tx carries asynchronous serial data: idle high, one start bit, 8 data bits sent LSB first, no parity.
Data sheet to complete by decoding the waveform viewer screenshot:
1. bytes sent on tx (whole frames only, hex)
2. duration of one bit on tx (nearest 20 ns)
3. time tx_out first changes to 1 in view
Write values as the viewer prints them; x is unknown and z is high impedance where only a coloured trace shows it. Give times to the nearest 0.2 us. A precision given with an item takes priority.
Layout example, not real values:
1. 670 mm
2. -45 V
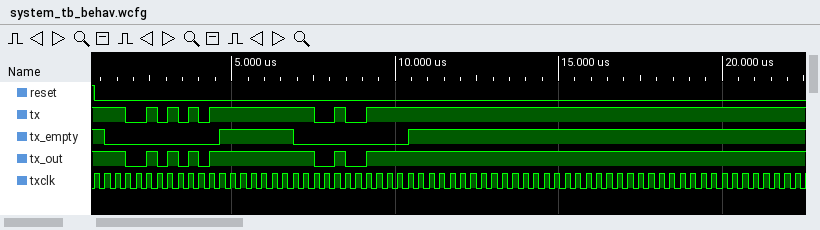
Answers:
1. AA, F2
2. 320 ns
3. 2.4 us
